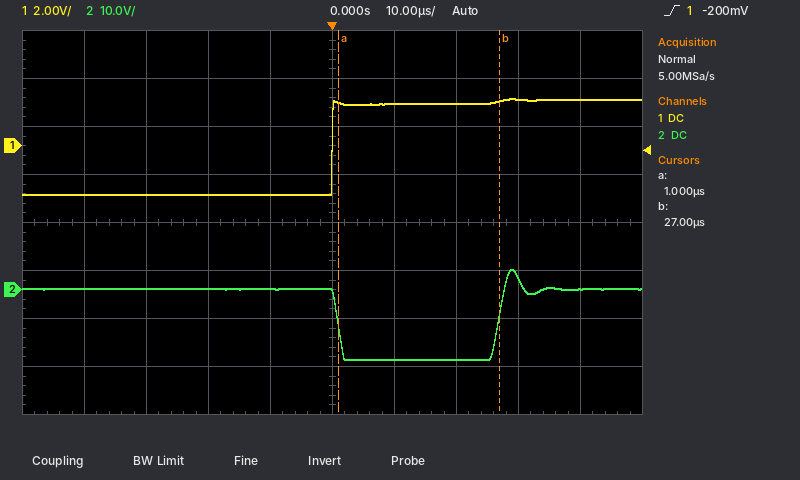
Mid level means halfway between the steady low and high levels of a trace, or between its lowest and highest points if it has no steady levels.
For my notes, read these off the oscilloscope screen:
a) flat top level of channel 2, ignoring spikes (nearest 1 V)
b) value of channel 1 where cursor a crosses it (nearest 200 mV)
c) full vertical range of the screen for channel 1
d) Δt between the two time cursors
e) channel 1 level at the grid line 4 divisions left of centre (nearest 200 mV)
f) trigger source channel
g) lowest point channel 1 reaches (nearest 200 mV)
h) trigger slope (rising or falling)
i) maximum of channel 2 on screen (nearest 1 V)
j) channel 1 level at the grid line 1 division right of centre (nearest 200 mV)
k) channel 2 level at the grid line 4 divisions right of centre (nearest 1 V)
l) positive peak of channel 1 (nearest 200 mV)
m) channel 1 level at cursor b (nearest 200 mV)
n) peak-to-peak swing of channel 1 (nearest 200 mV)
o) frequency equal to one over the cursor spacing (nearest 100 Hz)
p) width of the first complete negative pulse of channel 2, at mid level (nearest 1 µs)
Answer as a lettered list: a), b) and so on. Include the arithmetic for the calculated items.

a) 0 V
b) 1.8 V
c) 16 V
d) 27 µs − (1 µs) = 26 µs
e) -2.0 V
f) channel 1
g) -2.0 V
h) rising
i) 4 V
j) 1.8 V
k) 0 V
l) 2.0 V
m) 1.8 V
n) 2.0 V − (-2.0 V) = 4.0 V
o) 1 / 26 µs ≈ 38.5 kHz
p) 26 µs
